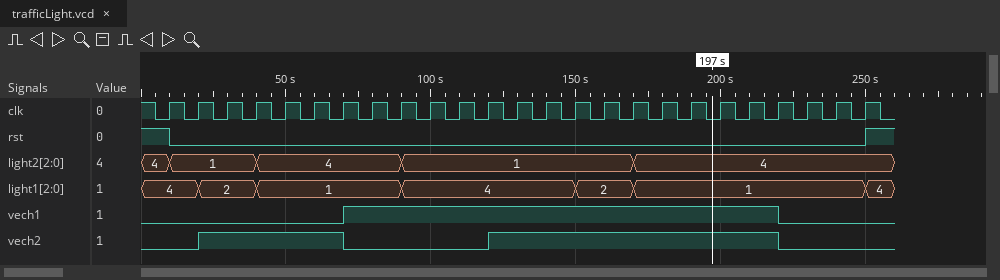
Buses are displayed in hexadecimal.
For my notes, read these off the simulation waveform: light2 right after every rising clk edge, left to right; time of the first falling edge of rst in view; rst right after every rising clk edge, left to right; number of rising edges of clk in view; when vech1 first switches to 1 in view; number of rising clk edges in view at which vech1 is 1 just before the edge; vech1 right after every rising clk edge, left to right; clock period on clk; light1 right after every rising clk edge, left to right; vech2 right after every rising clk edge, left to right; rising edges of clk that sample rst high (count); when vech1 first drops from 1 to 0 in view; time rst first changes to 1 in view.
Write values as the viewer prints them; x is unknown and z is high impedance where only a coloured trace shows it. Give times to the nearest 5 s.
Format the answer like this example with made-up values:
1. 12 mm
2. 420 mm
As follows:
1. 1, 1, 1, 4, 4, 4, 4, 4, 1, 1, 1, 1, 1, 1, 1, 1, 4, 4, 4, 4, 4, 4, 4, 4, 4
2. 10 s
3. 0 0 0 0 0 0 0 0 0 0 0 0 0 0 0 0 0 0 0 0 0 0 0 0 1
4. 25
5. 70 s
6. 15
7. 0 0 0 0 0 0 1 1 1 1 1 1 1 1 1 1 1 1 1 1 1 0 0 0 0
8. 10 s
9. 4, 2, 2, 1, 1, 1, 1, 1, 4, 4, 4, 4, 4, 4, 2, 2, 1, 1, 1, 1, 1, 1, 1, 1, 4
10. 0 1 1 1 1 1 0 0 0 0 0 1 1 1 1 1 1 1 1 1 1 0 0 0 0
11. 1
12. 220 s
13. 250 s
